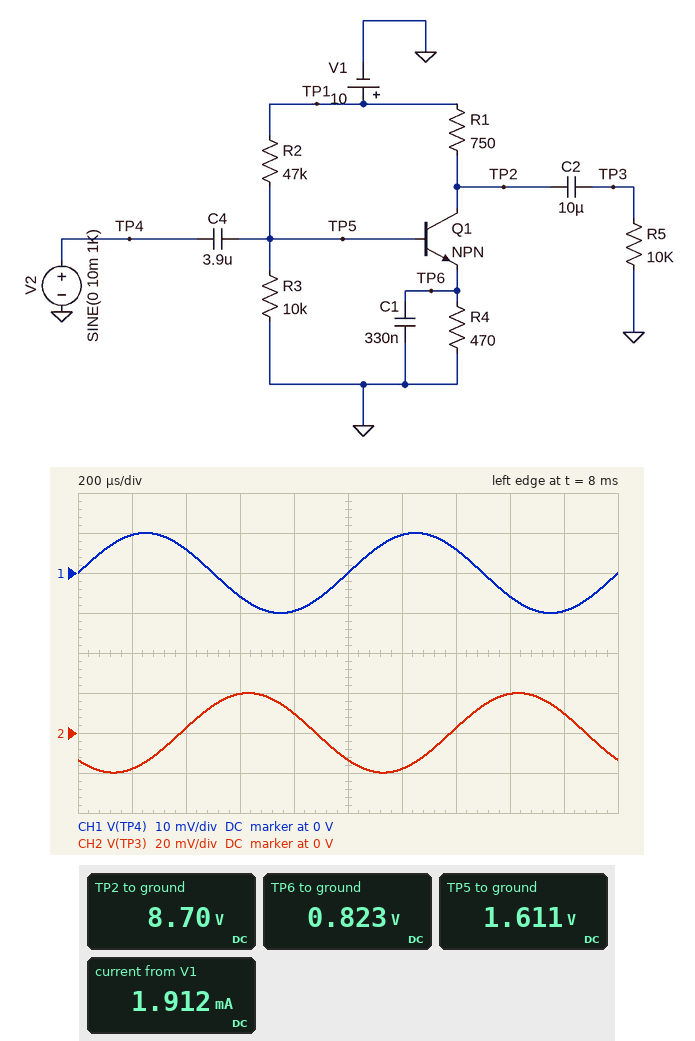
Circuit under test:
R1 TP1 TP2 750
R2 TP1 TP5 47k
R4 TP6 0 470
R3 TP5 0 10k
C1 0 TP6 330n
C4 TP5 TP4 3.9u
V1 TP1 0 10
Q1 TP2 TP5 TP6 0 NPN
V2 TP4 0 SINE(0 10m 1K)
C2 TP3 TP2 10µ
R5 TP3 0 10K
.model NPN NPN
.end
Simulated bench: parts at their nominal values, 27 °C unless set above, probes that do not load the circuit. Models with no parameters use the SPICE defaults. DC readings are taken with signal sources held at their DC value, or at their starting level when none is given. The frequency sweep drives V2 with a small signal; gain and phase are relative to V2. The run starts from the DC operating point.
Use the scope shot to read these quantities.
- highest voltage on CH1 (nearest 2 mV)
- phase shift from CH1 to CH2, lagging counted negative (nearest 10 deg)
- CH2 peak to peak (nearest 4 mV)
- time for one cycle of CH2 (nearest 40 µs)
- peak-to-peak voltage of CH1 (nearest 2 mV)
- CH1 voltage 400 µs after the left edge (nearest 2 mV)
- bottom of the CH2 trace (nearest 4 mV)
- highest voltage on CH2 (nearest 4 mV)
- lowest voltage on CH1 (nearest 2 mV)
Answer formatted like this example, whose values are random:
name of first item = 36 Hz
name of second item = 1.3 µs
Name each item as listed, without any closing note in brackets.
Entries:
highest voltage on CH1 = 10 mV
phase shift from CH1 to CH2, lagging counted negative = -140 deg
CH2 peak to peak = 40 mV
time for one cycle of CH2 = 1.00 ms
peak-to-peak voltage of CH1 = 20 mV
CH1 voltage 400 µs after the left edge = 6 mV
bottom of the CH2 trace = -20 mV
highest voltage on CH2 = 20 mV
lowest voltage on CH1 = -10 mV
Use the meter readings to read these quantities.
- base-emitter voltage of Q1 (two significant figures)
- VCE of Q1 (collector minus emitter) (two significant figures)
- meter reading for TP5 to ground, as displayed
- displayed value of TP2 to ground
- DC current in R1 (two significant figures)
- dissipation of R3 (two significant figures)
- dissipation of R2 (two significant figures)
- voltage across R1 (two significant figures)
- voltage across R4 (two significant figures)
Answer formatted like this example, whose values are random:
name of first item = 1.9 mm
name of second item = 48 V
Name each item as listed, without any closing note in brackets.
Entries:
base-emitter voltage of Q1 = 790 mV
VCE of Q1 (collector minus emitter) = 7.9 V
meter reading for TP5 to ground, as displayed = 1.611 V
displayed value of TP2 to ground = 8.70 V
DC current in R1 = 1.7 mA
dissipation of R3 = 260 µW
dissipation of R2 = 1.5 mW
voltage across R1 = 1.3 V
voltage across R4 = 820 mV
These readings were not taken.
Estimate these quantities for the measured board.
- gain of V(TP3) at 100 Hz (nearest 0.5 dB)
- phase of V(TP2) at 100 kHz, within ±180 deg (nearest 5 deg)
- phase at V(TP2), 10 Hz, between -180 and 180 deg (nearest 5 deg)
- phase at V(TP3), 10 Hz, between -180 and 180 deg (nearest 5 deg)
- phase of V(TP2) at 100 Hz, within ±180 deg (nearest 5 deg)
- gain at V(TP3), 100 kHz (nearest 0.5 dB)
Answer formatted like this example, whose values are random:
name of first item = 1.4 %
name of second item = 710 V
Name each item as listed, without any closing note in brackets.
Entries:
gain of V(TP3) at 100 Hz = 3.0 dB
phase of V(TP2) at 100 kHz, within ±180 deg = -160 deg
phase at V(TP2), 10 Hz, between -180 and 180 deg = -150 deg
phase at V(TP3), 10 Hz, between -180 and 180 deg = -140 deg
phase of V(TP2) at 100 Hz, within ±180 deg = -170 deg
gain at V(TP3), 100 kHz = 33.0 dB
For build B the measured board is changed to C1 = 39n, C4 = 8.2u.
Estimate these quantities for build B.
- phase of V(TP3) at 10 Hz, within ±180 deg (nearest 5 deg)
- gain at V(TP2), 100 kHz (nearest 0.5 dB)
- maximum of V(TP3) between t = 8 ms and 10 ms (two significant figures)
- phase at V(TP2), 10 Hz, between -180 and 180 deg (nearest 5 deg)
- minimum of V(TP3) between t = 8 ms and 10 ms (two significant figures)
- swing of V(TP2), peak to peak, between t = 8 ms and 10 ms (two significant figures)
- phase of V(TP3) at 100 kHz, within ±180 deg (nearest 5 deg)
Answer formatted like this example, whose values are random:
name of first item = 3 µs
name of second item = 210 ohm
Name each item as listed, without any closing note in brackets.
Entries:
phase of V(TP3) at 10 Hz, within ±180 deg = -155 deg
gain at V(TP2), 100 kHz = 24.0 dB
maximum of V(TP3) between t = 8 ms and 10 ms = 14 mV
phase at V(TP2), 10 Hz, between -180 and 180 deg = -165 deg
minimum of V(TP3) between t = 8 ms and 10 ms = -14 mV
swing of V(TP2), peak to peak, between t = 8 ms and 10 ms = 29 mV
phase of V(TP3) at 100 kHz, within ±180 deg = -115 deg
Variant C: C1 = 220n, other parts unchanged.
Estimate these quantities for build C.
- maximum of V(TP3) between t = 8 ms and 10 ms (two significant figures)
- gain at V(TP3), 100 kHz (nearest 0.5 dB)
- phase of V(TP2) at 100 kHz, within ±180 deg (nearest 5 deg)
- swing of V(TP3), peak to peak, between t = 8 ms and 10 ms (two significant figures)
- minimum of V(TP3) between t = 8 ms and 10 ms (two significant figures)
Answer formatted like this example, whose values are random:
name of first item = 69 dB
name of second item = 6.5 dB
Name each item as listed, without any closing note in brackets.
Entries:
maximum of V(TP3) between t = 8 ms and 10 ms = 17 mV
gain at V(TP3), 100 kHz = 32.5 dB
phase of V(TP2) at 100 kHz, within ±180 deg = -155 deg
swing of V(TP3), peak to peak, between t = 8 ms and 10 ms = 34 mV
minimum of V(TP3) between t = 8 ms and 10 ms = -17 mV
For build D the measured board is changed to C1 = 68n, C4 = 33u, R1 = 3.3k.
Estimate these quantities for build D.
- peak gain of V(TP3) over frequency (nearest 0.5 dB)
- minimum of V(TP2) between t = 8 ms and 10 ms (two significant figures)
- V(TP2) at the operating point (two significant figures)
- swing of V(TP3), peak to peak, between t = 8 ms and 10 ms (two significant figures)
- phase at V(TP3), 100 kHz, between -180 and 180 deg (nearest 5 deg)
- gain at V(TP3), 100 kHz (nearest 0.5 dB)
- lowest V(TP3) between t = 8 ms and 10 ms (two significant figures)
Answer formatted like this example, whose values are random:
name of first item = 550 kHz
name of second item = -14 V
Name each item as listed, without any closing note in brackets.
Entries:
peak gain of V(TP3) over frequency = 44.5 dB
minimum of V(TP2) between t = 8 ms and 10 ms = 4.2 V
V(TP2) at the operating point = 4.3 V
swing of V(TP3), peak to peak, between t = 8 ms and 10 ms = 100 mV
phase at V(TP3), 100 kHz, between -180 and 180 deg = -125 deg
gain at V(TP3), 100 kHz = 39.0 dB
lowest V(TP3) between t = 8 ms and 10 ms = -52 mV
